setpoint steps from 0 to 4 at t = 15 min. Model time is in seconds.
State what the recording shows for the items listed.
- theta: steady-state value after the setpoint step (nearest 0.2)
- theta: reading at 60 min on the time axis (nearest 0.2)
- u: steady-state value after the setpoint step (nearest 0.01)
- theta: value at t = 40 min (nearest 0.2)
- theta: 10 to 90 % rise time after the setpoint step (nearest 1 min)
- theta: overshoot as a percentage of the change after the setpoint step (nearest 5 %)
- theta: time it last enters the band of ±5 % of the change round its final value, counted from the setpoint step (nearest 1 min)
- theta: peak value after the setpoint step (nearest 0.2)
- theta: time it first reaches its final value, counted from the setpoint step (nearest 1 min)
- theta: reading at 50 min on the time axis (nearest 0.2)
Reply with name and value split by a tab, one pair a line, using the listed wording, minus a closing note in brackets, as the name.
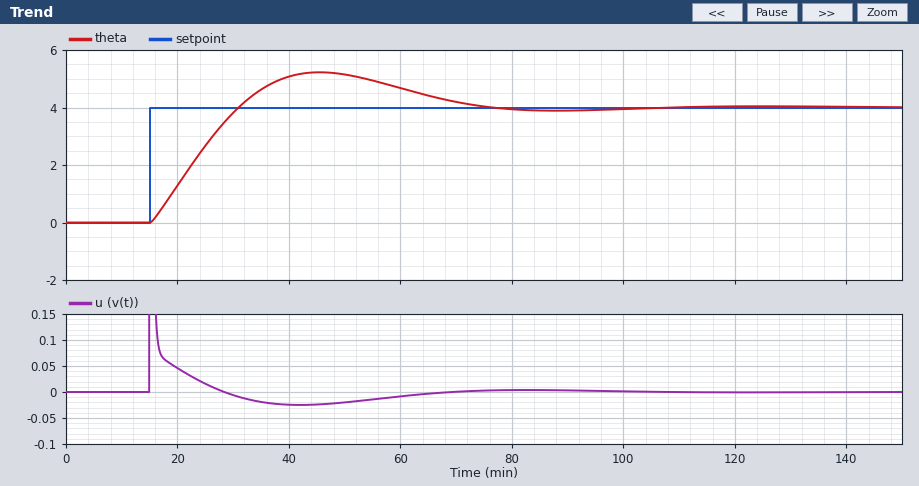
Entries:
theta: steady-state value after the setpoint step	4.0
theta: reading at 60 min on the time axis	4.6
u: steady-state value after the setpoint step	0.00
theta: value at t = 40 min	5.0
theta: 10 to 90 % rise time after the setpoint step	12 min
theta: overshoot as a percentage of the change after the setpoint step	30 %
theta: time it last enters the band of ±5 % of the change round its final value, counted from the setpoint step	55 min
theta: peak value after the setpoint step	5.2
theta: time it first reaches its final value, counted from the setpoint step	16 min
theta: reading at 50 min on the time axis	5.2
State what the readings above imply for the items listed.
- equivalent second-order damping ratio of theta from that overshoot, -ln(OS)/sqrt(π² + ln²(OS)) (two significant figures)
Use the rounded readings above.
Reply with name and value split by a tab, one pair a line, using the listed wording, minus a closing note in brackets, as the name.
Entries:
equivalent second-order damping ratio of theta from that overshoot, -ln(OS)/sqrt(π² + ln²(OS))	0.36
